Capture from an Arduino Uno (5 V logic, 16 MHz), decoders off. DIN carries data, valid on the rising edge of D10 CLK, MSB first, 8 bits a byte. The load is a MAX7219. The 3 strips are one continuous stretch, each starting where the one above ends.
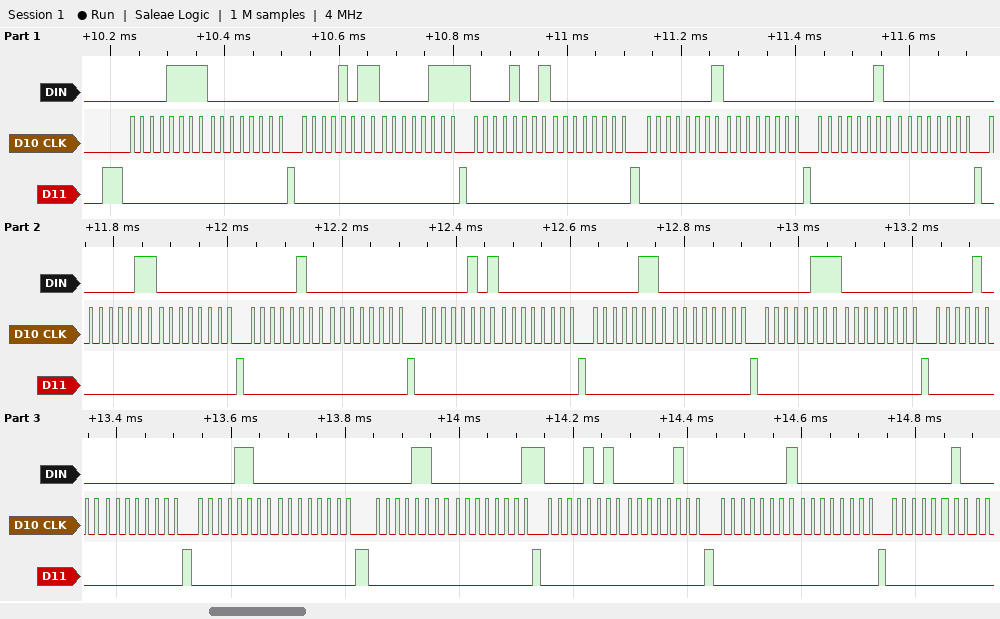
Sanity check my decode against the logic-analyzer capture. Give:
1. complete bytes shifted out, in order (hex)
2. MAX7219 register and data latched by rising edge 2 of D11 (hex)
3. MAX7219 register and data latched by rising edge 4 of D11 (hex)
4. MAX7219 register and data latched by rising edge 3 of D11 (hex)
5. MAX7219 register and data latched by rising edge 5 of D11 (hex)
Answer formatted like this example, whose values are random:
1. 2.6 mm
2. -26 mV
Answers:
1. 0F 00 0B 07 09 00 01 00 02 00 03 00 04 00 05 00 06 00 07 00 08 00 0C 00 0C 01 0A 04 01 00 02
2. register 0xF, data 0x00
3. register 0x9, data 0x00
4. register 0xB, data 0x07
5. register 0x1, data 0x00
